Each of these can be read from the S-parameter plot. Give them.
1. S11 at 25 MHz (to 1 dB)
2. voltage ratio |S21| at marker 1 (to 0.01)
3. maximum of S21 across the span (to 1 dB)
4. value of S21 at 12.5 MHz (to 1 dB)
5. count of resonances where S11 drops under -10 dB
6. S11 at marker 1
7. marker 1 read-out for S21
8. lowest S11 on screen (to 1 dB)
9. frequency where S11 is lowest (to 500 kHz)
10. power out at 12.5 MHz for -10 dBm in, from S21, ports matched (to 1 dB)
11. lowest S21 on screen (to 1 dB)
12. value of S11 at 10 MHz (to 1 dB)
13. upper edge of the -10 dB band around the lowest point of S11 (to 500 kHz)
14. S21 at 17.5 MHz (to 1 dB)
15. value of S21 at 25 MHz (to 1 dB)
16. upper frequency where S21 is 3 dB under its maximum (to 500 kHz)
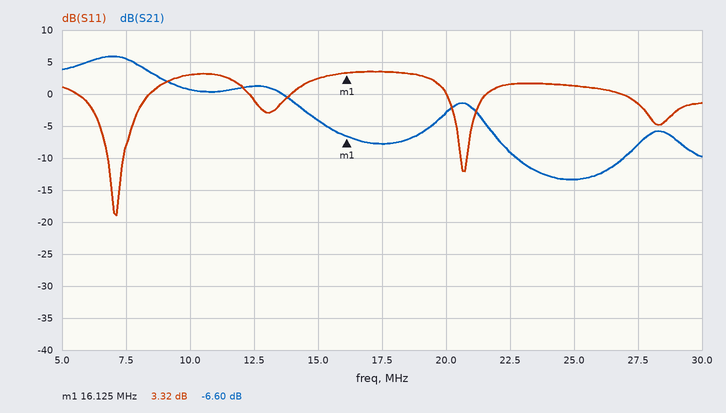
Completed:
1 dB
0.47
6 dB
1 dB
2
3.32 dB
-6.60 dB
-19 dB
7.0 MHz
-9 dBm
-13 dB
3 dB
7.5 MHz
-8 dB
-13 dB
8.5 MHz
